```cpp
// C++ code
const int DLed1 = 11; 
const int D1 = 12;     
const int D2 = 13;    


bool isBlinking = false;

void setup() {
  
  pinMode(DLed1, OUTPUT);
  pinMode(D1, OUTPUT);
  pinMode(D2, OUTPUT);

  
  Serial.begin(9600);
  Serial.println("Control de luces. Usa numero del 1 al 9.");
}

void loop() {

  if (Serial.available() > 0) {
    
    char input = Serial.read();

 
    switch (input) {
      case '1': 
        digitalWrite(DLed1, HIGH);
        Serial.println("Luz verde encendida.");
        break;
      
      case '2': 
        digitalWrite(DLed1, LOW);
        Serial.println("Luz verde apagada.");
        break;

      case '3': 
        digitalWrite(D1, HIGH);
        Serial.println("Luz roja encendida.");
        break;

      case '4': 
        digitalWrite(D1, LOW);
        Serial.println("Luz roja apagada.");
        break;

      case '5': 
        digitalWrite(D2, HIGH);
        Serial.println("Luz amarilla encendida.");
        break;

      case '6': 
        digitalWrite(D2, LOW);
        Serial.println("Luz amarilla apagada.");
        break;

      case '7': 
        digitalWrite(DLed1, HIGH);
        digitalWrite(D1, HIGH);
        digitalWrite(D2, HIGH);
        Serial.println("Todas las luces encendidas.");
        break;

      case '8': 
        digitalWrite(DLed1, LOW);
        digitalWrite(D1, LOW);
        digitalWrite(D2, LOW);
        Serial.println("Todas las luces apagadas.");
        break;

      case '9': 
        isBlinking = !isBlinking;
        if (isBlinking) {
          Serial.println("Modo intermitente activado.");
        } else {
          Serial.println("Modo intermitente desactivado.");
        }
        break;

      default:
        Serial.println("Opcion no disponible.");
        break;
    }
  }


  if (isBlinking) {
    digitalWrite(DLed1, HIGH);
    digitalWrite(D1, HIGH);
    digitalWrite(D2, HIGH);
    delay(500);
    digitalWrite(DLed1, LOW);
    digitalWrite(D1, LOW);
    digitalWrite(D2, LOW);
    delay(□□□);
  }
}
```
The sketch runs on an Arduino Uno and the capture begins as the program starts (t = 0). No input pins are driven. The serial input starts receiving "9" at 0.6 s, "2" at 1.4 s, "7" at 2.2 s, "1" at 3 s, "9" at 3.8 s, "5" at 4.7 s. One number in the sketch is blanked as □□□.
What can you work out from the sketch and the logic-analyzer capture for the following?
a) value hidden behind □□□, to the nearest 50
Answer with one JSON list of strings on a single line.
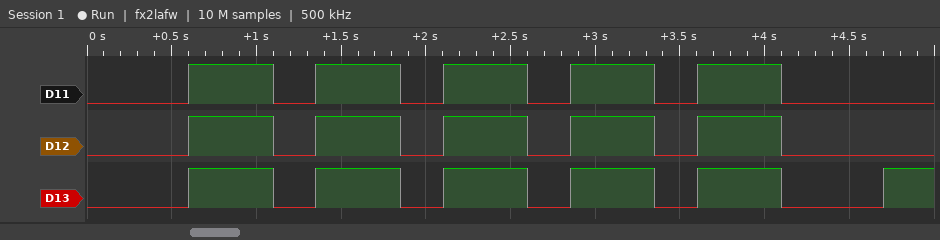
["250"]
